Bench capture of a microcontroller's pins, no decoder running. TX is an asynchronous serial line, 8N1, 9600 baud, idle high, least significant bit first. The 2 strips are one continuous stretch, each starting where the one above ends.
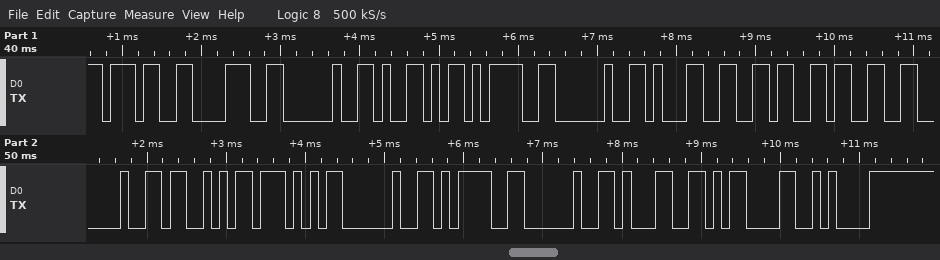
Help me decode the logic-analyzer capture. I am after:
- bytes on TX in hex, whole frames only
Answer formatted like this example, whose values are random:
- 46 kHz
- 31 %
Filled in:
- 37 38 20 59 3D 20 31 36 33 20 53 57 20 3D 20 31 0D 0A
